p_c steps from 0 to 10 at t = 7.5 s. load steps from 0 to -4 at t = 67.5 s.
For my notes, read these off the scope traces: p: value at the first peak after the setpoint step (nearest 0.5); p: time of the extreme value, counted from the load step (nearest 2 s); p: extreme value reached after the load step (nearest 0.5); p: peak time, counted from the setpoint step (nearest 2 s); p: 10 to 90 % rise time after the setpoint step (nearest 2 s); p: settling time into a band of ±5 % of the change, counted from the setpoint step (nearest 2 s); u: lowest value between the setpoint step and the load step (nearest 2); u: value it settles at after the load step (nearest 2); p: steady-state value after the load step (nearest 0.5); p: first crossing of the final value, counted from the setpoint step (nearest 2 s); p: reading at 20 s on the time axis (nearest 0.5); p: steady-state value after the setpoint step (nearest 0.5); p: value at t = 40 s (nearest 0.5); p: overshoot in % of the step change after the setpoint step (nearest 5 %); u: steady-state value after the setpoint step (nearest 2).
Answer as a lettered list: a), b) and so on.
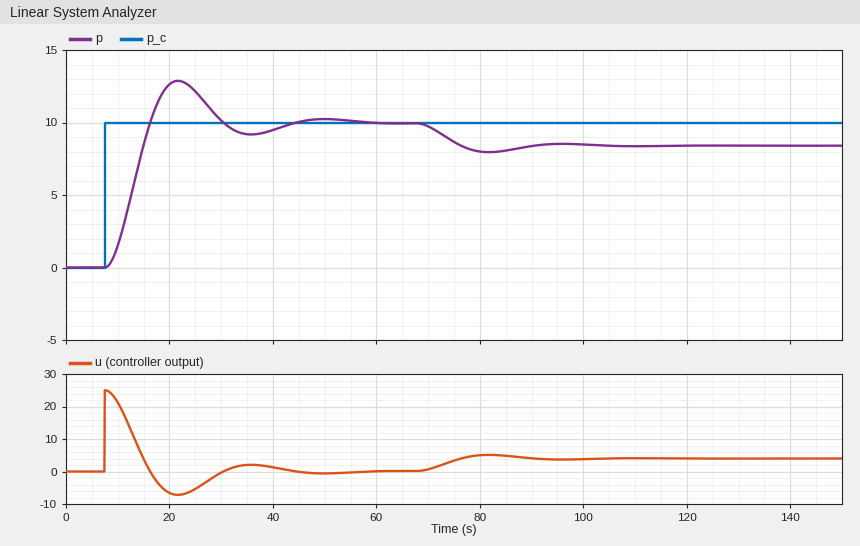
a) 13.0
b) 14 s
c) 8.0
d) 14 s
e) 6 s
f) 32 s
g) -8
h) 4
i) 8.5
j) 8 s
k) 12.5
l) 10.0
m) 9.5
n) 30 %
o) 0
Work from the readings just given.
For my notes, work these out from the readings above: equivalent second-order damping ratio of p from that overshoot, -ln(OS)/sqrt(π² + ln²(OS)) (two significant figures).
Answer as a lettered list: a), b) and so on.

a) 0.36
